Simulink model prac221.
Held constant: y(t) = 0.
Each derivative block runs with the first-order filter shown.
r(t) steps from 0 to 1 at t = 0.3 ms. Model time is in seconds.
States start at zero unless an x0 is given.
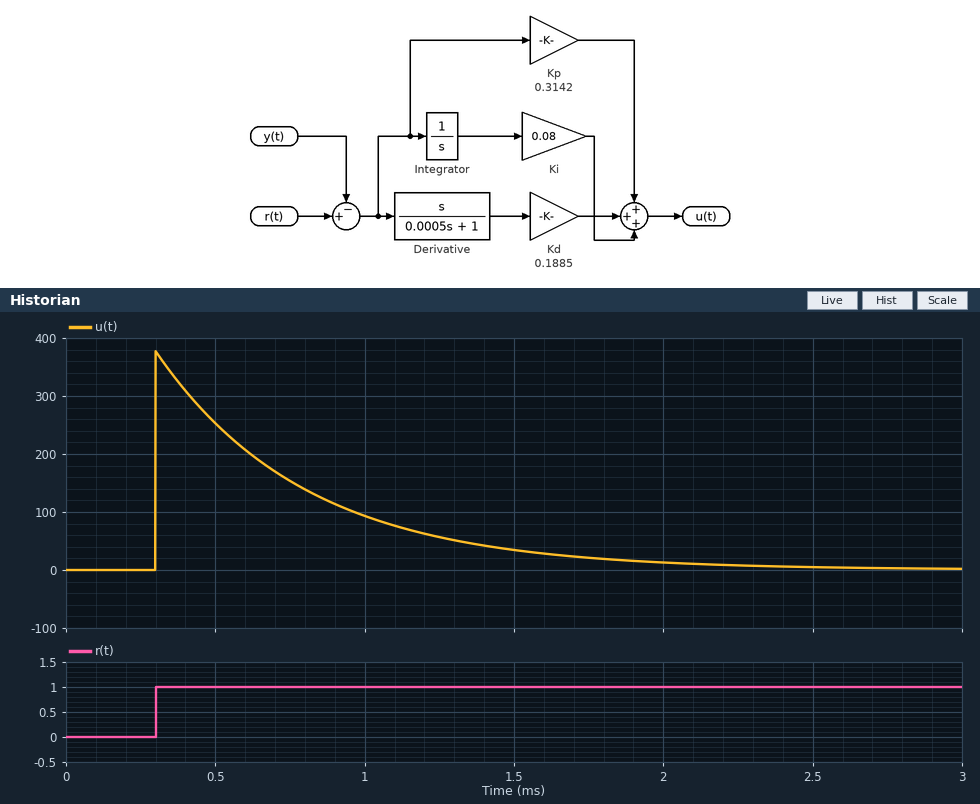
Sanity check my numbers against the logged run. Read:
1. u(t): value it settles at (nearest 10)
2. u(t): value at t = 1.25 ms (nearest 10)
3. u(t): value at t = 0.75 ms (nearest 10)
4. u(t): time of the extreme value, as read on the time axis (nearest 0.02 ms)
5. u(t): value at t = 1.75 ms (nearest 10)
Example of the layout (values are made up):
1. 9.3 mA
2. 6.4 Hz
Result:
1. 0
2. 60
3. 150
4. 0.30 ms
5. 20
